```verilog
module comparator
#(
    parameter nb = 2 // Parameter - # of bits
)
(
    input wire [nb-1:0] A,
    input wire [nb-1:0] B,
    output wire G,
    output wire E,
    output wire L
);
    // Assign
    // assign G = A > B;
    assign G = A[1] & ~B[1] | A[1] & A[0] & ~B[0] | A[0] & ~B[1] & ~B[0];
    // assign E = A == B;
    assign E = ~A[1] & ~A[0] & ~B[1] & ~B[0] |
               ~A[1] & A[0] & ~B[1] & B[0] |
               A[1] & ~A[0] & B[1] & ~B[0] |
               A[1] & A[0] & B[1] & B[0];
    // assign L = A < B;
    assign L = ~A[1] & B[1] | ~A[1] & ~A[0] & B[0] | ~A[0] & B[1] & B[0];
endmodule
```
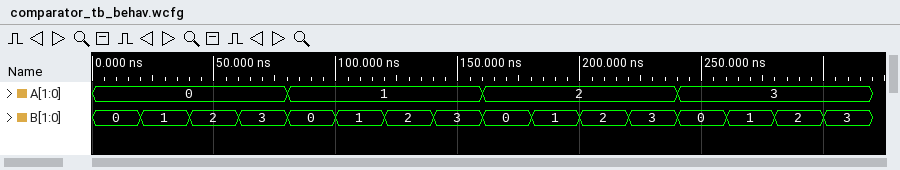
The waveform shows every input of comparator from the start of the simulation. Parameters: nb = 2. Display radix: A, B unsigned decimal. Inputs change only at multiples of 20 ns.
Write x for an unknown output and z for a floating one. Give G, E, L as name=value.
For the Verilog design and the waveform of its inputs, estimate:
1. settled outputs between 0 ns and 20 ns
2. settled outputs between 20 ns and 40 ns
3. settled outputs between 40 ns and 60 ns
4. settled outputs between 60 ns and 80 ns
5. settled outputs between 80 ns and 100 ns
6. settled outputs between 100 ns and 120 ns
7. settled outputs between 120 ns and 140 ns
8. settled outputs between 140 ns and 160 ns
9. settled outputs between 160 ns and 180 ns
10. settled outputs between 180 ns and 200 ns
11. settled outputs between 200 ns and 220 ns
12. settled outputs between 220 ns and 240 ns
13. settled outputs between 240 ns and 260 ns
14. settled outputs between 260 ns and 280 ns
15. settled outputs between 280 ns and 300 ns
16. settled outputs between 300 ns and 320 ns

G=0, E=1, L=0
G=0, E=0, L=1
G=0, E=0, L=1
G=0, E=0, L=1
G=1, E=0, L=0
G=0, E=1, L=0
G=0, E=0, L=1
G=0, E=0, L=1
G=1, E=0, L=0
G=1, E=0, L=0
G=0, E=1, L=0
G=0, E=0, L=1
G=1, E=0, L=0
G=1, E=0, L=0
G=1, E=0, L=0
G=0, E=1, L=0
